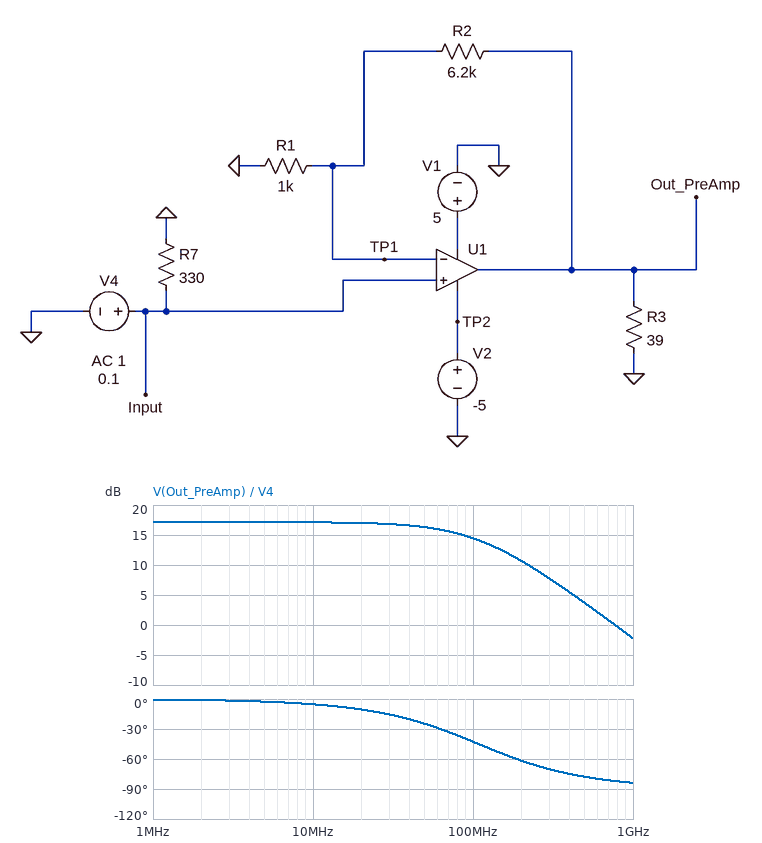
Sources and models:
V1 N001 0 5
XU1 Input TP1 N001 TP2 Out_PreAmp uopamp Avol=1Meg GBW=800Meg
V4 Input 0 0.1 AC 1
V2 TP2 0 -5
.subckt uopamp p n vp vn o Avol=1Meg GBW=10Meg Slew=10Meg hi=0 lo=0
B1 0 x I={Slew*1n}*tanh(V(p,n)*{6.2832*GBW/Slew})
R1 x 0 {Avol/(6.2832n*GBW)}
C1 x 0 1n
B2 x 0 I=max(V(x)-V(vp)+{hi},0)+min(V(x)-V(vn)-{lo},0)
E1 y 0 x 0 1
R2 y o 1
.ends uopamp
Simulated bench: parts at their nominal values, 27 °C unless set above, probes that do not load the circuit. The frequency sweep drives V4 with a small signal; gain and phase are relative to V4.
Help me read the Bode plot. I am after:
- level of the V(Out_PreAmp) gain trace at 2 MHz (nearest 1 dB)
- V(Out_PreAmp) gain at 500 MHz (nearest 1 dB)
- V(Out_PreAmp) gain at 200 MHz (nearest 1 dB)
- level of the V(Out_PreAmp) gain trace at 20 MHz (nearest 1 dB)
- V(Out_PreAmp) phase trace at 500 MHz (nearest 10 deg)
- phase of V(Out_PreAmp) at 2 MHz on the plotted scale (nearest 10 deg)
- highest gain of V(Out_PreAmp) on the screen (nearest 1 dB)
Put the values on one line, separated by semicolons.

17 dB; 4 dB; 11 dB; 17 dB; -80 deg; 0 deg; 17 dB
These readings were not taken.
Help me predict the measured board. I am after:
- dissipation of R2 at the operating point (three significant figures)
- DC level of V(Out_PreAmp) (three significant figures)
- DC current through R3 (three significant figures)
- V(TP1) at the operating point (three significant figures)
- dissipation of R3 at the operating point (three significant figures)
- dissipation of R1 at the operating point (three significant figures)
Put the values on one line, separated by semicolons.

62.0 µW; 720 mV; 18.5 mA; 100 mV; 13.3 mW; 10.0 µW
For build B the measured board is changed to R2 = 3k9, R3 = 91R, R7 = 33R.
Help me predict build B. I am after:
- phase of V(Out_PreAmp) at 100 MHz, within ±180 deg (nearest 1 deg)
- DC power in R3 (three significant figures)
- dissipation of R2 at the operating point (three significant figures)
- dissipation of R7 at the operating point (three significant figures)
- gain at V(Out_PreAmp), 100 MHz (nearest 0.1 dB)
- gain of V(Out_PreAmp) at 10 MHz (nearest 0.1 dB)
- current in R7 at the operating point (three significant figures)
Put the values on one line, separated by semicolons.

-32 deg; 2.64 mW; 39.0 µW; 303 µW; 12.4 dB; 13.8 dB; 3.03 mA
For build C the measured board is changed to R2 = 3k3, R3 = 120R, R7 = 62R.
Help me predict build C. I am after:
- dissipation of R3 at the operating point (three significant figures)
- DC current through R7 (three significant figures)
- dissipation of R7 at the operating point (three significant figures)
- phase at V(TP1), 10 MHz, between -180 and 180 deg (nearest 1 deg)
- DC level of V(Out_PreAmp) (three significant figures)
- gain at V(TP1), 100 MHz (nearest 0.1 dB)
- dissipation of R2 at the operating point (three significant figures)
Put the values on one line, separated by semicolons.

1.54 mW; 1.61 mA; 161 µW; -3 deg; 430 mV; -1.1 dB; 33.0 µW
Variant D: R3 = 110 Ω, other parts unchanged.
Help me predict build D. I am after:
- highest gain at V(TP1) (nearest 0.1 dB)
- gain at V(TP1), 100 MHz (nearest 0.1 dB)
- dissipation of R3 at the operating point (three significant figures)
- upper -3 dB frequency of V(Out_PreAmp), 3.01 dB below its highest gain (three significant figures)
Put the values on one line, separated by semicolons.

0 dB; -2.6 dB; 4.71 mW; 110 MHz
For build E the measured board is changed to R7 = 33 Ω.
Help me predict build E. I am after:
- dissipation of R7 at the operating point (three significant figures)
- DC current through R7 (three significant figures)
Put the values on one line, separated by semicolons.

303 µW; 3.03 mA
